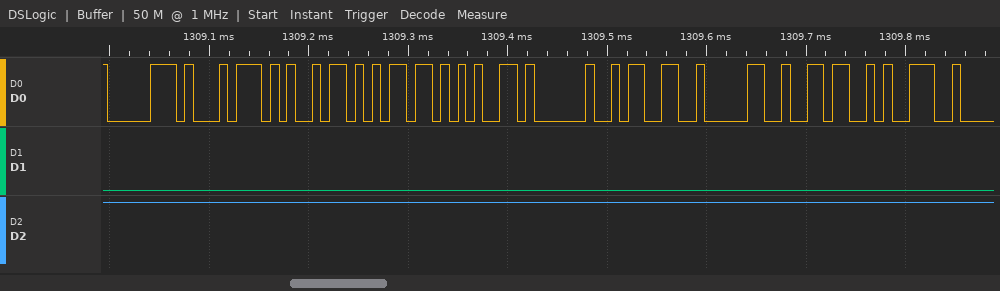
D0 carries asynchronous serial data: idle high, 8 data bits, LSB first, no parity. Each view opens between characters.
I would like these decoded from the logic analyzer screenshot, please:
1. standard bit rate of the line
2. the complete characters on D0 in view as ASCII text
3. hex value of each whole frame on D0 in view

115200 baud
"ptime 3069"
70, 74, 69, 6D, 65, 20, 33, 30, 36, 39
